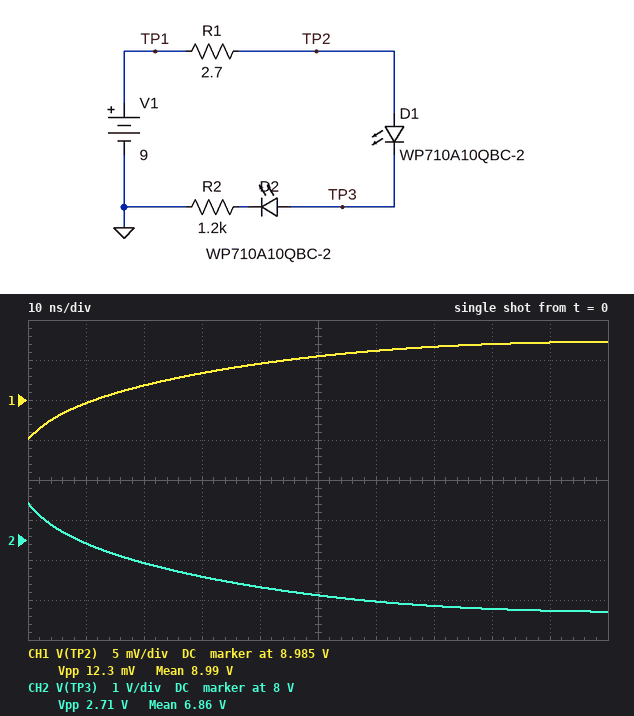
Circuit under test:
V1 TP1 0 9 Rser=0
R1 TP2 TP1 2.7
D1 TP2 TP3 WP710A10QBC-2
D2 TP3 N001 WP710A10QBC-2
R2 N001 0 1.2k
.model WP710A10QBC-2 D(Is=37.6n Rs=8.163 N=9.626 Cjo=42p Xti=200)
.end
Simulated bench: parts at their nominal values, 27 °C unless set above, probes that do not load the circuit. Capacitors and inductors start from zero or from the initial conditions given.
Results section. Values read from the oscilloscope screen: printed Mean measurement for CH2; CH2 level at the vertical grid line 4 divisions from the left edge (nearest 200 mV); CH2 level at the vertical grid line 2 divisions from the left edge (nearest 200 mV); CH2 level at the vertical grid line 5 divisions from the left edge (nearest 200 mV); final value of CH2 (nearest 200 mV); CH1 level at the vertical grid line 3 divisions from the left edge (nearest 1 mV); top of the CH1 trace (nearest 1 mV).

6.86 V
6.8 V
7.4 V
6.6 V
6.2 V
8.988 V
8.992 V
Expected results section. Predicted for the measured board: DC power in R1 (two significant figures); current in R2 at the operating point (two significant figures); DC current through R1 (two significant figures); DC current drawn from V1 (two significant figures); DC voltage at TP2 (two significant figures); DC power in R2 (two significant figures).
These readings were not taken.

21 µW
2.8 mA
2.8 mA
2.8 mA
9.0 V
9.4 mW
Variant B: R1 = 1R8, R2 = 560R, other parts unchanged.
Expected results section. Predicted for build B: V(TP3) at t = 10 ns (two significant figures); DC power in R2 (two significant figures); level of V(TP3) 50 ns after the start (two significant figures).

7.3 V
16 mW
6.0 V
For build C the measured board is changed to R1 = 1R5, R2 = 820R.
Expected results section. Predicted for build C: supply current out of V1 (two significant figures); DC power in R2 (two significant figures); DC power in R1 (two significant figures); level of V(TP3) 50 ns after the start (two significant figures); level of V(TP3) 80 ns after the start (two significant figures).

3.9 mA
12 mW
23 µW
6.3 V
6.1 V
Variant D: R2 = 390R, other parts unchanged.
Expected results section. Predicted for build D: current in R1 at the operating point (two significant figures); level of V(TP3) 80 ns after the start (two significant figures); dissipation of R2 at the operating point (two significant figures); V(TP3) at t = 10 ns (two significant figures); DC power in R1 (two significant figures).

7.2 mA
5.9 V
20 mW
7.0 V
140 µW
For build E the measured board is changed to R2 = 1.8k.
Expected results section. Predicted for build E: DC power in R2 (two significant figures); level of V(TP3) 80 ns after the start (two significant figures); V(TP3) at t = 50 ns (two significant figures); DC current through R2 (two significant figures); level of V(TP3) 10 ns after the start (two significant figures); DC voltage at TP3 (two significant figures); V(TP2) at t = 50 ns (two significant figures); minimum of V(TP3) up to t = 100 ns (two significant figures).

7.0 mW
6.6 V
7.0 V
2.0 mA
8.2 V
6.3 V
9.0 V
6.4 V
